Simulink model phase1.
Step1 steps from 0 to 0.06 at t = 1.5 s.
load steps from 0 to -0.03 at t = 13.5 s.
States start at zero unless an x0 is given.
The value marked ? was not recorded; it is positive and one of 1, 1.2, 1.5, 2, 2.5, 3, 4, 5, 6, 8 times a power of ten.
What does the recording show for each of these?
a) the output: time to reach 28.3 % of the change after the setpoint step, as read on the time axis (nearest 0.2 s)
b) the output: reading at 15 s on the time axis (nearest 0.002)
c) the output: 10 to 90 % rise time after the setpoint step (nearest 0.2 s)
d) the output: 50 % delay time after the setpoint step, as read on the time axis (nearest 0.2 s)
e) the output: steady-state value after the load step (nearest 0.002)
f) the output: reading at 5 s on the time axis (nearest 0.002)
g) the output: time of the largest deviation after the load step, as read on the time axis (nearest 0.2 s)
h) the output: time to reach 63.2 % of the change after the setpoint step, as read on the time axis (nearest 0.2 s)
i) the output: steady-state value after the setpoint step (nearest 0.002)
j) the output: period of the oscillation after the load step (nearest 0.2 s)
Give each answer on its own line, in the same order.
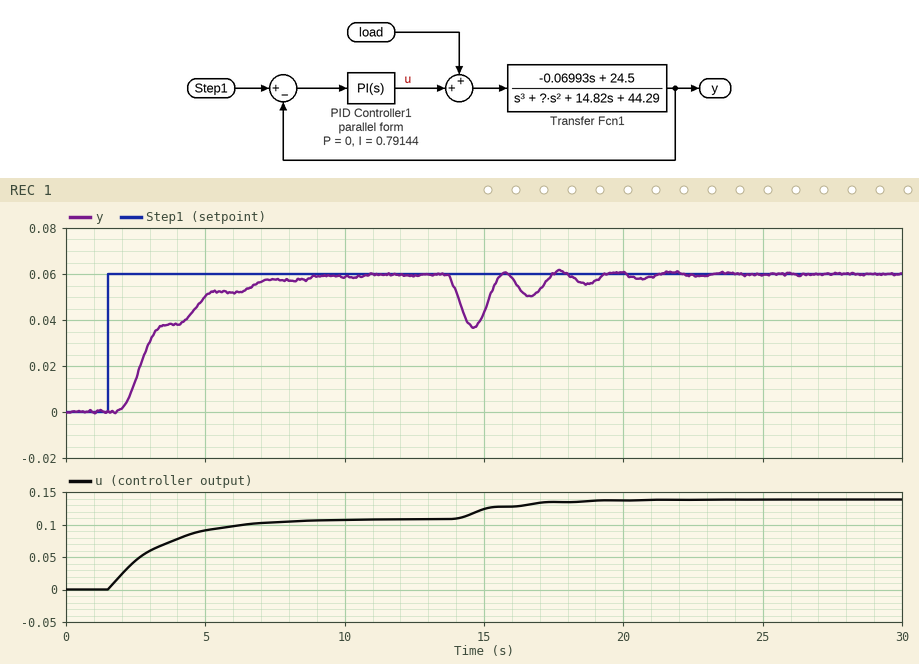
2.6 s
0.044
4.4 s
3.0 s
0.060
0.050
14.6 s
3.6 s
0.060
2.0 s
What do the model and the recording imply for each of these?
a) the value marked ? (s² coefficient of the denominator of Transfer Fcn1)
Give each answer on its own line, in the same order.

5
